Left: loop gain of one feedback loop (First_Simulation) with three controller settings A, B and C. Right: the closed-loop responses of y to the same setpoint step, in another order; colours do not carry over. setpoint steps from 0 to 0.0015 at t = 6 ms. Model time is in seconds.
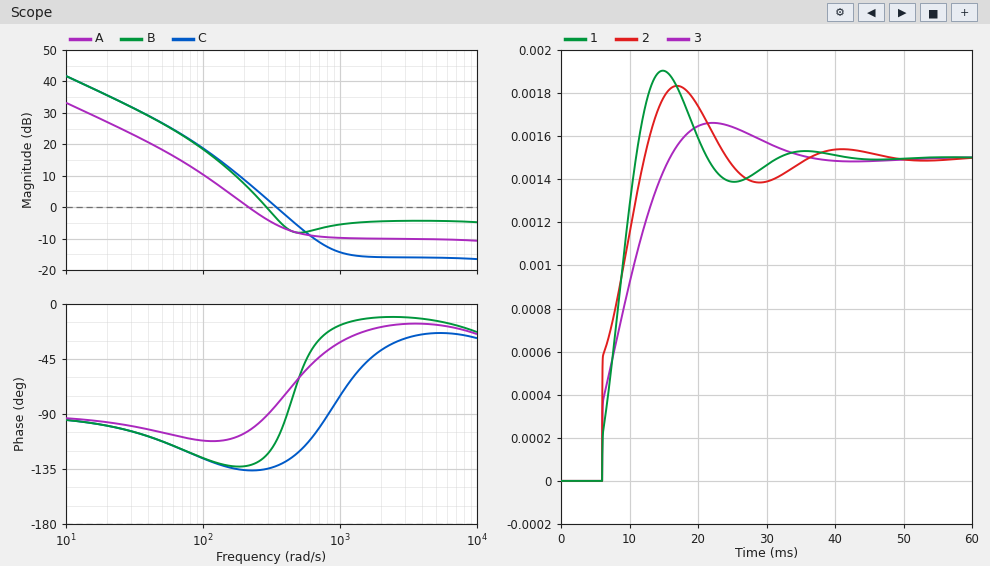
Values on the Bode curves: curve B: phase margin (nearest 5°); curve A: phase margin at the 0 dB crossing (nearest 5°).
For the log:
55°
75°
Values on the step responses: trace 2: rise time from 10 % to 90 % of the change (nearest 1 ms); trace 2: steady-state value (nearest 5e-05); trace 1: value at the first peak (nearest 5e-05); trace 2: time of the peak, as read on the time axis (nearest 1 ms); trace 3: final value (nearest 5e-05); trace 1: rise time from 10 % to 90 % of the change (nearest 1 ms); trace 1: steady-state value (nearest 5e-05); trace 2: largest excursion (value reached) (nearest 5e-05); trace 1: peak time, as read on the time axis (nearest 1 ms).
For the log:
5 ms
0.00150
0.00190
17 ms
0.00150
4 ms
0.00150
0.00185
15 ms
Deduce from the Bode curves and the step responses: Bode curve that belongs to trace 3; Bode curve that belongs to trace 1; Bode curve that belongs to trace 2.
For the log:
A
C
B
